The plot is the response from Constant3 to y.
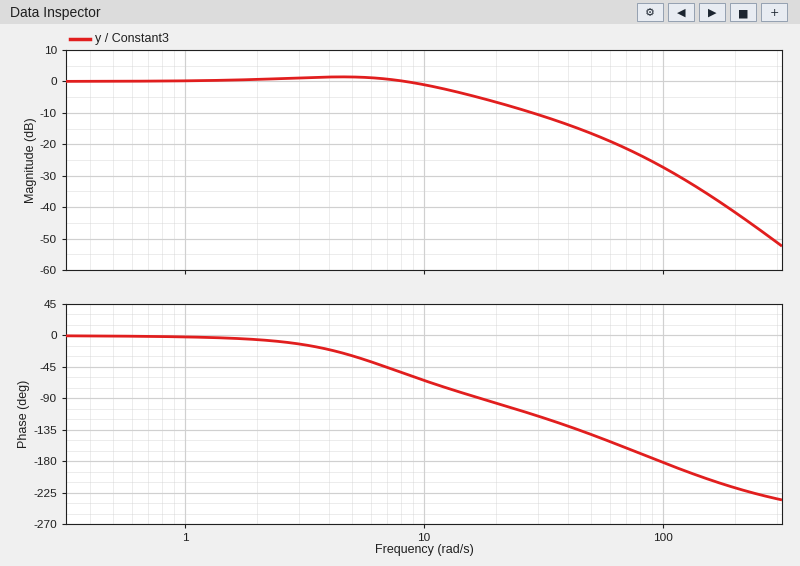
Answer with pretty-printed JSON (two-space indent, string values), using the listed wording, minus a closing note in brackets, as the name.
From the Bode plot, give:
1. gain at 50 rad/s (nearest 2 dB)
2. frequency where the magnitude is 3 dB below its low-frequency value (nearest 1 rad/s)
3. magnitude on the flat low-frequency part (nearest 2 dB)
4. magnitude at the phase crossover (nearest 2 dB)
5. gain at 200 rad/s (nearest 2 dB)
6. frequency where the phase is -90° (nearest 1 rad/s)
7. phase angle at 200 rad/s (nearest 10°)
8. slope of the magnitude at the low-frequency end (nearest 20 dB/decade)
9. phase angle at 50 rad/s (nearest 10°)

{
  "gain at 50 rad/s": "-16 dB",
  "frequency where the magnitude is 3 dB below its low-frequency value": "13 rad/s",
  "magnitude on the flat low-frequency part": "0 dB",
  "magnitude at the phase crossover": "-26 dB",
  "gain at 200 rad/s": "-42 dB",
  "frequency where the phase is -90°": "17 rad/s",
  "phase angle at 200 rad/s": "-220°",
  "slope of the magnitude at the low-frequency end": "0 dB/decade",
  "phase angle at 50 rad/s": "-140°"
}
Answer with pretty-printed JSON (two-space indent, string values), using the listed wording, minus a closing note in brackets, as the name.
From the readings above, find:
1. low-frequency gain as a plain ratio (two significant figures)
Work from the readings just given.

{
  "low-frequency gain as a plain ratio": "1.0"
}
